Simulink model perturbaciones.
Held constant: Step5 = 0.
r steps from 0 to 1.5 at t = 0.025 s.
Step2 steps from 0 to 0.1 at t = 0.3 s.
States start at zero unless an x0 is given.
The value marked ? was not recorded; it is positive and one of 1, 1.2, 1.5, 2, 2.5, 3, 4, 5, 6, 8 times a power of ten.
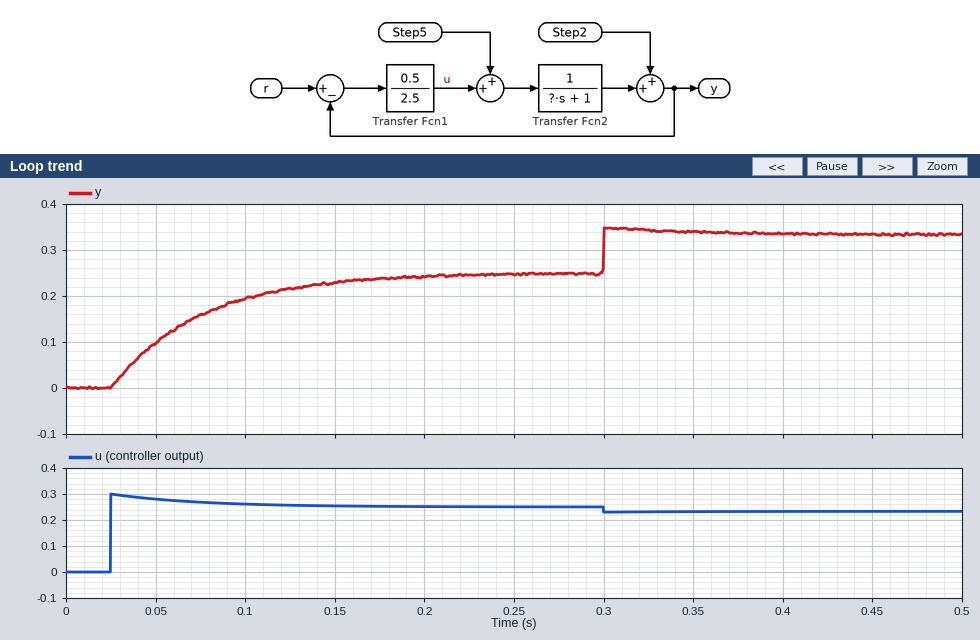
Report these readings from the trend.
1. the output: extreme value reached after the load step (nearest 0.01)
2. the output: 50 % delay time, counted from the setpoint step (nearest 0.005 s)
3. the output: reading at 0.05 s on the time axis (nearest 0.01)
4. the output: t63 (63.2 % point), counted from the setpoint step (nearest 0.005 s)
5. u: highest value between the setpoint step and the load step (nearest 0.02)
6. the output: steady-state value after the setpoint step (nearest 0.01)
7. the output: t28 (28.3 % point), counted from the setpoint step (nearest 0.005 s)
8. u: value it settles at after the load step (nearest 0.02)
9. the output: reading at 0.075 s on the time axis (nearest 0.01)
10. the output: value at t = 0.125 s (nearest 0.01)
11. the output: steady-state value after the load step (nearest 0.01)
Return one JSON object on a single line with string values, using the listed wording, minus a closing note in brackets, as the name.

{"the output: extreme value reached after the load step": "0.35", "the output: 50 % delay time, counted from the setpoint step": "0.035 s", "the output: reading at 0.05 s on the time axis": "0.10", "the output: t63 (63.2 % point), counted from the setpoint step": "0.050 s", "u: highest value between the setpoint step and the load step": "0.30", "the output: steady-state value after the setpoint step": "0.25", "the output: t28 (28.3 % point), counted from the setpoint step": "0.015 s", "u: value it settles at after the load step": "0.24", "the output: reading at 0.075 s on the time axis": "0.16", "the output: value at t = 0.125 s": "0.22", "the output: steady-state value after the load step": "0.33"}
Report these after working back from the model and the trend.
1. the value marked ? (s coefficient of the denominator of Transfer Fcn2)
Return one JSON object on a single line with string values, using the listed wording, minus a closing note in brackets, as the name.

{"the value marked ?": "0.06"}
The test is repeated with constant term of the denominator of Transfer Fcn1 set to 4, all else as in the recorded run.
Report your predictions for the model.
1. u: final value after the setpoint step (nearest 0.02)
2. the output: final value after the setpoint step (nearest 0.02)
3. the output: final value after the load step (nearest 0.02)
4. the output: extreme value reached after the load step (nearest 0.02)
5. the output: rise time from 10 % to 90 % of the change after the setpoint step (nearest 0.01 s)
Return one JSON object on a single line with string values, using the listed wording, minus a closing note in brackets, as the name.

{"u: final value after the setpoint step": "0.16", "the output: final value after the setpoint step": "0.16", "the output: final value after the load step": "0.26", "the output: extreme value reached after the load step": "0.26", "the output: rise time from 10 % to 90 % of the change after the setpoint step": "0.12 s"}
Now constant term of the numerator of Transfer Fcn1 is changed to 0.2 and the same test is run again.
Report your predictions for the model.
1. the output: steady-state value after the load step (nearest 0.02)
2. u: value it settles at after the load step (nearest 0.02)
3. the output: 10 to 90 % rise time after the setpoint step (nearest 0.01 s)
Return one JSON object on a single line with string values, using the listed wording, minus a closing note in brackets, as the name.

{"the output: steady-state value after the load step": "0.20", "u: value it settles at after the load step": "0.10", "the output: 10 to 90 % rise time after the setpoint step": "0.12 s"}
